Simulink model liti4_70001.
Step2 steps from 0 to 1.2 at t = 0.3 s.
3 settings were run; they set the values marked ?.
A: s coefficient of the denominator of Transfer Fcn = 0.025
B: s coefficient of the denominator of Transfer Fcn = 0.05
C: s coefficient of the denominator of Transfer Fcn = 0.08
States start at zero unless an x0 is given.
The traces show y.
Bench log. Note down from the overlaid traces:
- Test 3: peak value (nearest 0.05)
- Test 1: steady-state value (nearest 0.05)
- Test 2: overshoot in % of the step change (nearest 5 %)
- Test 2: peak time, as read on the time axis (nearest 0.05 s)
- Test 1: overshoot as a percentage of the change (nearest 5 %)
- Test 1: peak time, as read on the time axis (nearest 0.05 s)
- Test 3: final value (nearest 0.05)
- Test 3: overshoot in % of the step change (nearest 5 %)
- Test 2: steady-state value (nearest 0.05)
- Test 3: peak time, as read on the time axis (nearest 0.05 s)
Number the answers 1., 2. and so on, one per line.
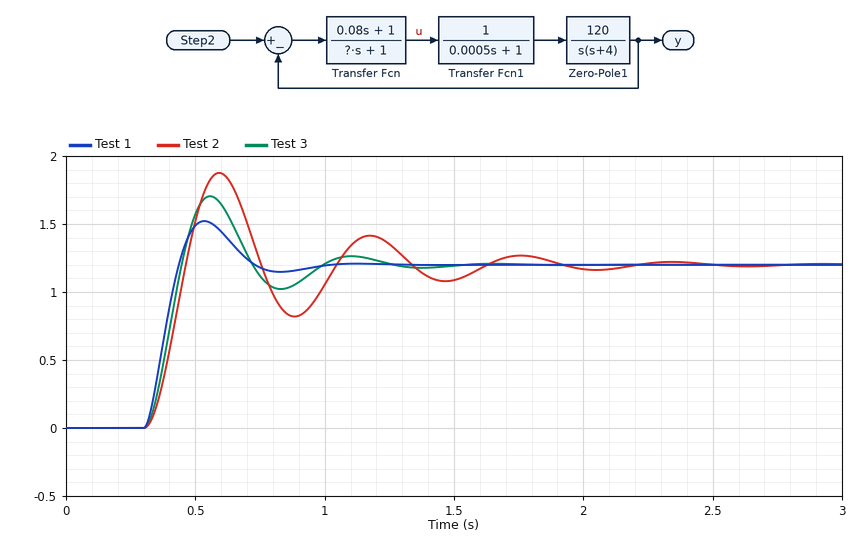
1. 1.70
2. 1.20
3. 55 %
4. 0.60 s
5. 25 %
6. 0.55 s
7. 1.20
8. 40 %
9. 1.20
10. 0.55 s
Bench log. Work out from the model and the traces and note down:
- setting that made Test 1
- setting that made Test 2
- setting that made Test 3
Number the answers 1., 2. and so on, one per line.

1. A
2. C
3. B
